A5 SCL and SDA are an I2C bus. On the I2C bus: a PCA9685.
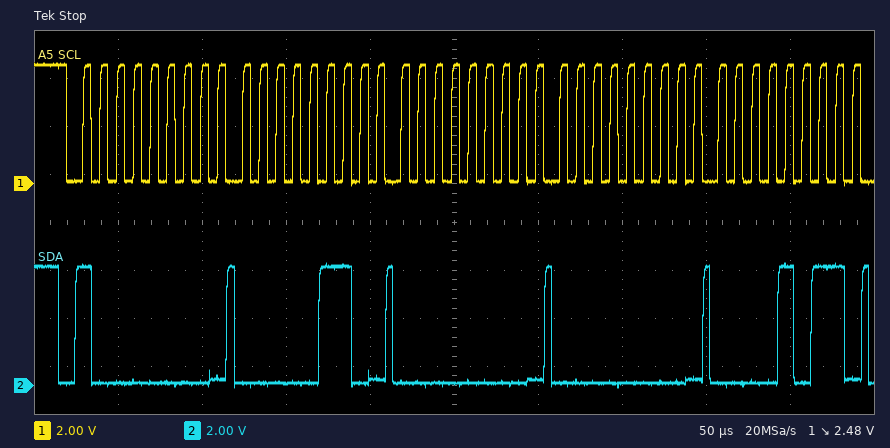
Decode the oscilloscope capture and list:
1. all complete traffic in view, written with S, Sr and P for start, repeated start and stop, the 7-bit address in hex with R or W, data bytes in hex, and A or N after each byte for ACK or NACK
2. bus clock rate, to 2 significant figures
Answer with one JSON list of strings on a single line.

["S 40W A 06 A 00 A 00 A 0B A", "100 kHz"]
